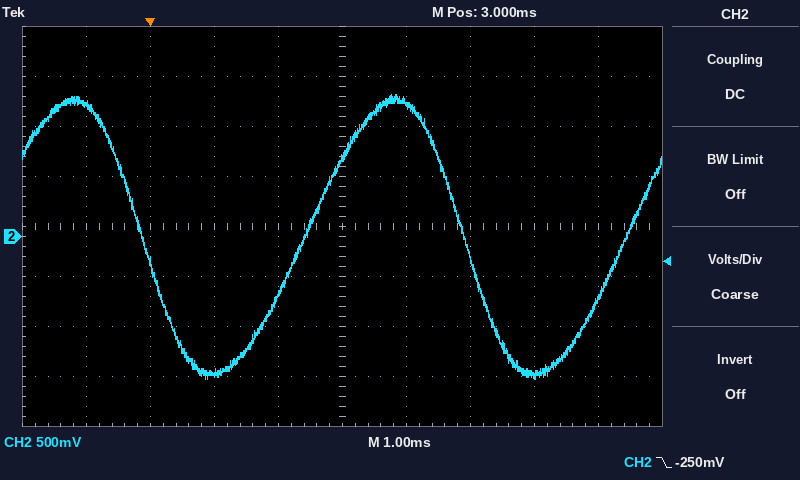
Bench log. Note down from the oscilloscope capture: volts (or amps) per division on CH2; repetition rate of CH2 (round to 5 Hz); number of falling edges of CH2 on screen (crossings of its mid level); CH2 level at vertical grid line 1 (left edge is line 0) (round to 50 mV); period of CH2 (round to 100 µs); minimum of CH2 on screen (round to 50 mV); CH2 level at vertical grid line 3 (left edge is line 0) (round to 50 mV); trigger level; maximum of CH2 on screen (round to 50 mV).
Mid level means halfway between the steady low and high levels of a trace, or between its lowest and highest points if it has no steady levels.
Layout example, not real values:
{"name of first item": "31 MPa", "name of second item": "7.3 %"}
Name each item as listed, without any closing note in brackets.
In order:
{"volts (or amps) per division on CH2": "500 mV", "repetition rate of CH2": "200 Hz", "number of falling edges of CH2 on screen": "2", "CH2 level at vertical grid line 1 (left edge is line 0)": "1.30 V", "period of CH2": "5.0 ms", "minimum of CH2 on screen": "-1.40 V", "CH2 level at vertical grid line 3 (left edge is line 0)": "-1.35 V", "trigger level": "-250 mV", "maximum of CH2 on screen": "1.40 V"}
